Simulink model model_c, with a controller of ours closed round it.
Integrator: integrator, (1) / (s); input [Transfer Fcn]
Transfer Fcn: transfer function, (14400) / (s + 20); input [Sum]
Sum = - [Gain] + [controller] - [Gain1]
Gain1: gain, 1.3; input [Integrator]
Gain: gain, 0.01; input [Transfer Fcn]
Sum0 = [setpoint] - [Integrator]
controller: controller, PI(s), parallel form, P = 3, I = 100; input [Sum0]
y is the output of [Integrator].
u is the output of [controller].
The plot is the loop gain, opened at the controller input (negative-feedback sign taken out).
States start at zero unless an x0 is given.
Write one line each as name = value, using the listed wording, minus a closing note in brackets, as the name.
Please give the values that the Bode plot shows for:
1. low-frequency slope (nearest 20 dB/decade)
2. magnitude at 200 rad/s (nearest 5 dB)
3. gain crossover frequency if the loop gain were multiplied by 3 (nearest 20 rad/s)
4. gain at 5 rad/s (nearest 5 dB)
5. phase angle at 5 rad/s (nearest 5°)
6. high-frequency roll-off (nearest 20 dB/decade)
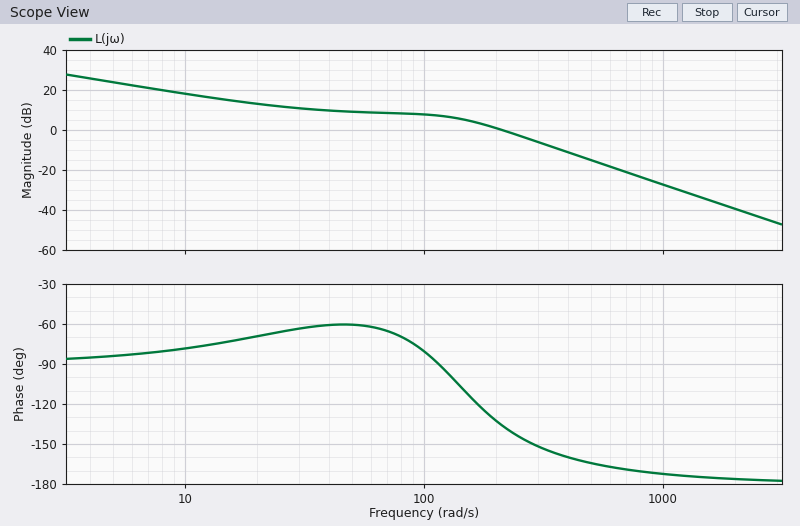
low-frequency slope = -20 dB/decade
magnitude at 200 rad/s = 0 dB
gain crossover frequency if the loop gain were multiplied by 3 = 360 rad/s
gain at 5 rad/s = 25 dB
phase angle at 5 rad/s = -85°
high-frequency roll-off = -40 dB/decade
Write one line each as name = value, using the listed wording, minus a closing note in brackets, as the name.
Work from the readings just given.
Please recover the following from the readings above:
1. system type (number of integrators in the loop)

system type = 1
